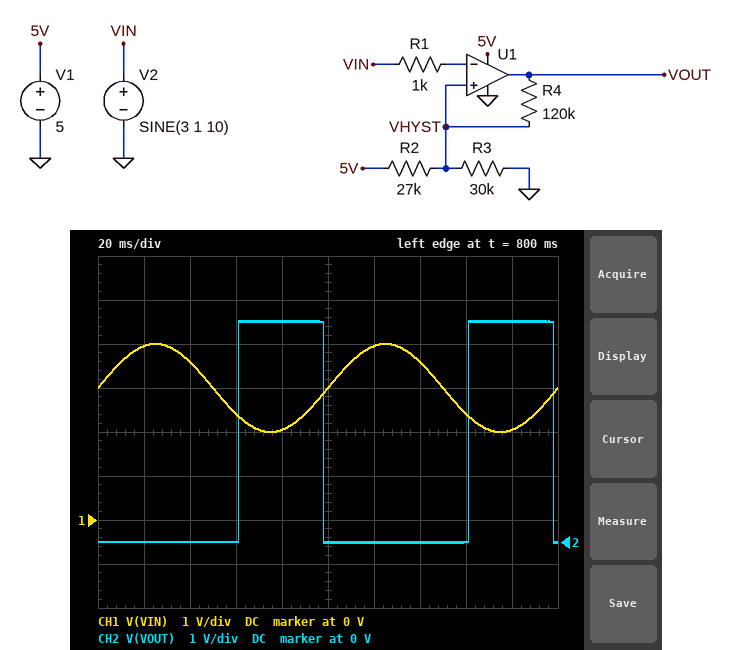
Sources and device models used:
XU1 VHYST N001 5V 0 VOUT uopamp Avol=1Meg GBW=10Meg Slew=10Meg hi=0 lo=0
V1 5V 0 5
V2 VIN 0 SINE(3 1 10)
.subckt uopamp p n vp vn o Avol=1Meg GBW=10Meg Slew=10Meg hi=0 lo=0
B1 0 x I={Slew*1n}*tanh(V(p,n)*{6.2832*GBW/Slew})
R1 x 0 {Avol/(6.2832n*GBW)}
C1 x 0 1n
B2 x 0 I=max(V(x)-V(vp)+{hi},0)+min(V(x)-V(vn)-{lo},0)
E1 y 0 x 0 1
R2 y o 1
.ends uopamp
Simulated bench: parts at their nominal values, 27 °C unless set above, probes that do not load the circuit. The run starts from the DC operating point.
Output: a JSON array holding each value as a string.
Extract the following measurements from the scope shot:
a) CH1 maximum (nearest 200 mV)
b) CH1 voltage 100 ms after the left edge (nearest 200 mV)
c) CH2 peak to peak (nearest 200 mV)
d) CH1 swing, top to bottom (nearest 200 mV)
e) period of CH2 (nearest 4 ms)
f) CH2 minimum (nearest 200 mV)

["4.0 V", "3.0 V", "5.0 V", "2.0 V", "100 ms", "0 V"]
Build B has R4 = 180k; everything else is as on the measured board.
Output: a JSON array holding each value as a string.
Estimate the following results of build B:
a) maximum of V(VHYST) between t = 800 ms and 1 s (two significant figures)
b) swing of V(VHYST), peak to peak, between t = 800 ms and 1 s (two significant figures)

["2.8 V", "370 mV"]
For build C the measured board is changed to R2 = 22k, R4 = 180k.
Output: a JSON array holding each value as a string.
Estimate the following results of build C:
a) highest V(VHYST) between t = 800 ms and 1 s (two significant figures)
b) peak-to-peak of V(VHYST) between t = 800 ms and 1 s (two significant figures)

["3.0 V", "330 mV"]
